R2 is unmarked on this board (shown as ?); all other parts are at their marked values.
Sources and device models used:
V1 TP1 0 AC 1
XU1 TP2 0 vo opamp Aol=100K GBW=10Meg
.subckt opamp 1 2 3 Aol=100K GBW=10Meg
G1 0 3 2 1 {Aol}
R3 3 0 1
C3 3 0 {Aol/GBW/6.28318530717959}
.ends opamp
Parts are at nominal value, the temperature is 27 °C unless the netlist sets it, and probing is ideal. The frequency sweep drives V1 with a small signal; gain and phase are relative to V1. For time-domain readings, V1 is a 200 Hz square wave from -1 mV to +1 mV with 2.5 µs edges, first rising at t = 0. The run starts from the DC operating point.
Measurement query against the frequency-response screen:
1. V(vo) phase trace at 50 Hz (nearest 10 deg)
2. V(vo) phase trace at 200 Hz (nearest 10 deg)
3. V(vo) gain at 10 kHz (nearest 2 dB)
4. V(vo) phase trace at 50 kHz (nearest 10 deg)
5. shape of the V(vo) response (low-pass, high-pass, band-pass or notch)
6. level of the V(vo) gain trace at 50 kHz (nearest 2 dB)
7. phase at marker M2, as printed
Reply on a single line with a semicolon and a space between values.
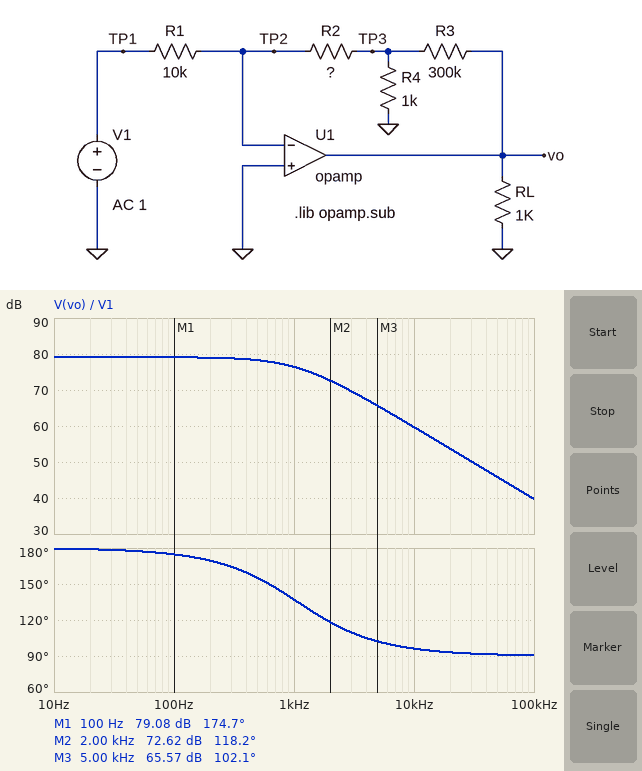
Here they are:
180 deg; 170 deg; 60 dB; 90 deg; low-pass; 46 dB; 118.2 deg
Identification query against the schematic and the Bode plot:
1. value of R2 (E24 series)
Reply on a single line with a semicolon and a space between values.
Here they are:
330 kΩ
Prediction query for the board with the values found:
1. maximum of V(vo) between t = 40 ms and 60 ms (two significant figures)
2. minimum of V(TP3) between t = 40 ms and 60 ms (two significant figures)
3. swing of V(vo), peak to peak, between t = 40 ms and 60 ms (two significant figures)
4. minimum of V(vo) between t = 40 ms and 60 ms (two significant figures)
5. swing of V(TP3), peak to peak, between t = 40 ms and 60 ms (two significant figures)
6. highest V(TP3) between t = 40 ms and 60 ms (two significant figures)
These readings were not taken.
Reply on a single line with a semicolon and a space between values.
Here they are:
9.0 V; -30 mV; 18 V; -9.0 V; 60 mV; 30 mV
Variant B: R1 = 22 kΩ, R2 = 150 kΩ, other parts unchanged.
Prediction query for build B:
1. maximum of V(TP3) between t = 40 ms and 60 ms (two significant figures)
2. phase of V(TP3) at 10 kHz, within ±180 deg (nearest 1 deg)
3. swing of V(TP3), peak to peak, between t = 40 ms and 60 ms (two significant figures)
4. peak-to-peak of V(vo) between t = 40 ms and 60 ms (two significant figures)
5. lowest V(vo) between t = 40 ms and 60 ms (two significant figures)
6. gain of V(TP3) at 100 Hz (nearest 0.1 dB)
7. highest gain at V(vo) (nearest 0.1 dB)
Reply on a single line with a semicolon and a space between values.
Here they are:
6.7 mV; 113 deg; 13 mV; 4.0 V; -2.0 V; 16.5 dB; 66.1 dB
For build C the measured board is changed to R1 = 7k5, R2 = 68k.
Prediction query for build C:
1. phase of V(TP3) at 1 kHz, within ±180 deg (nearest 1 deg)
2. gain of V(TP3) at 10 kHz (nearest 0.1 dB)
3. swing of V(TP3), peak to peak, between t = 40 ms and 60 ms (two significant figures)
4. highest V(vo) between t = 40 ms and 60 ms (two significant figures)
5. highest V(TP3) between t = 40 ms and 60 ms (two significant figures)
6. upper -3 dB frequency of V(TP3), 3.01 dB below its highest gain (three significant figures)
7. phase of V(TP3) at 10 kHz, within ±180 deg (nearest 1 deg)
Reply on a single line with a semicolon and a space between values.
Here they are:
163 deg; 8.9 dB; 18 mV; 2.7 V; 8.8 mV; 3.36 kHz; 108 deg
